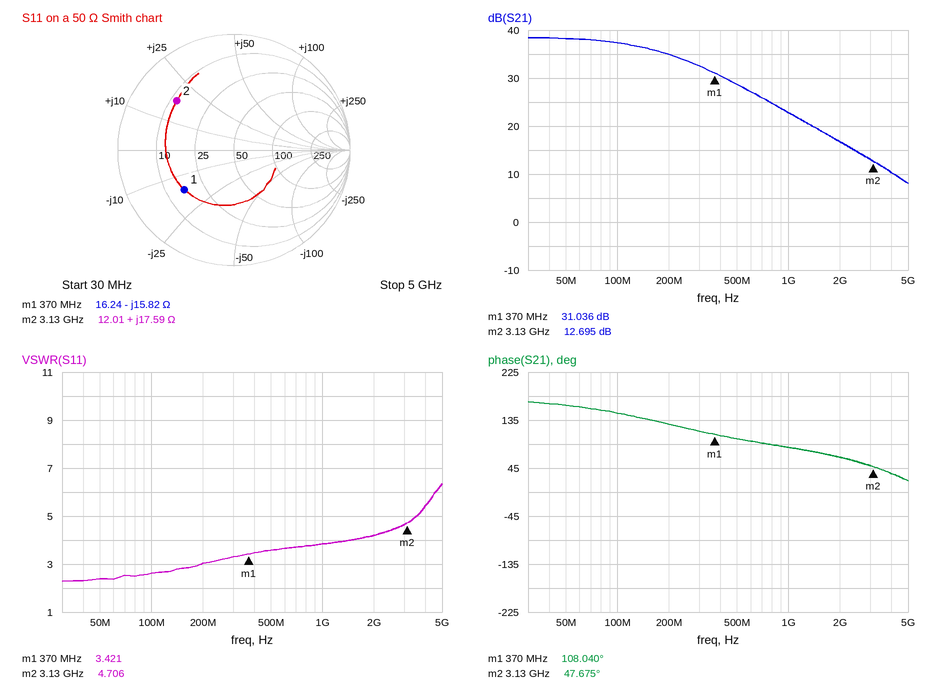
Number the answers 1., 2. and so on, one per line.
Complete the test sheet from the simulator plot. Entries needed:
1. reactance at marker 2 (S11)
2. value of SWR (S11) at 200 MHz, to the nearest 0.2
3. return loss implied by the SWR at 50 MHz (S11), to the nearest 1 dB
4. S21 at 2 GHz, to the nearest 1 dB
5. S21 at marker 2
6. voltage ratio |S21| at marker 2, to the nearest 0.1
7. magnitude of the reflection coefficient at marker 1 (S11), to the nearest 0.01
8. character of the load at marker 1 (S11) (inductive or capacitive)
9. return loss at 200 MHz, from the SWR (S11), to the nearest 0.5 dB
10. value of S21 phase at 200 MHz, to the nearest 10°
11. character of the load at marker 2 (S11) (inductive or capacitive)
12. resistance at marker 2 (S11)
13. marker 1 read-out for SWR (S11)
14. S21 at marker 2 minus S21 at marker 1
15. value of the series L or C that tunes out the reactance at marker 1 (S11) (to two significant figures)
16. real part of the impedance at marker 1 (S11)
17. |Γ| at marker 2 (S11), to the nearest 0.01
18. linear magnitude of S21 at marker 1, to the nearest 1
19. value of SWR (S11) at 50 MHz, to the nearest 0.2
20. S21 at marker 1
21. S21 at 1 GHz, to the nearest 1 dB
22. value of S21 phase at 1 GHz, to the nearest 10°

1. +17.59 Ω
2. 3.0
3. 8 dB
4. 17 dB
5. 12.695 dB
6. 4.3
7. 0.55
8. capacitive
9. 6.0 dB
10. 130°
11. inductive
12. 12.01 Ω
13. 3.421
14. -18.341 dB
15. 6.8 nH
16. 16.24 Ω
17. 0.65
18. 36
19. 2.4
20. 31.036 dB
21. 23 dB
22. 80°
